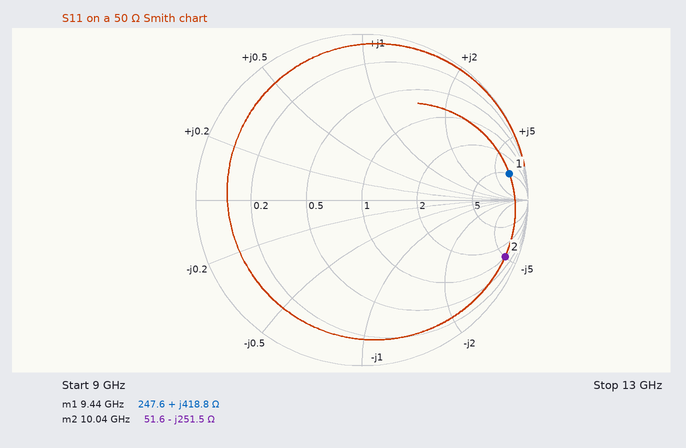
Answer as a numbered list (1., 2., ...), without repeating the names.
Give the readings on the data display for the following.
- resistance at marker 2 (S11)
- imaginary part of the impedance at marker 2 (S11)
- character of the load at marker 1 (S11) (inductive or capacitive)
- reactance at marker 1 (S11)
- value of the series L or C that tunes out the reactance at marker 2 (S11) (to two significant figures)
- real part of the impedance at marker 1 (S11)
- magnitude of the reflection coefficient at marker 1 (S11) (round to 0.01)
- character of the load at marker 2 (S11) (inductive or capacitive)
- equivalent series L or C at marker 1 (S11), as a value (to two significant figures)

1. 51.6 Ω
2. -251.5 Ω
3. inductive
4. +418.8 Ω
5. 4.0 nH
6. 247.6 Ω
7. 0.90
8. capacitive
9. 7.1 nH
